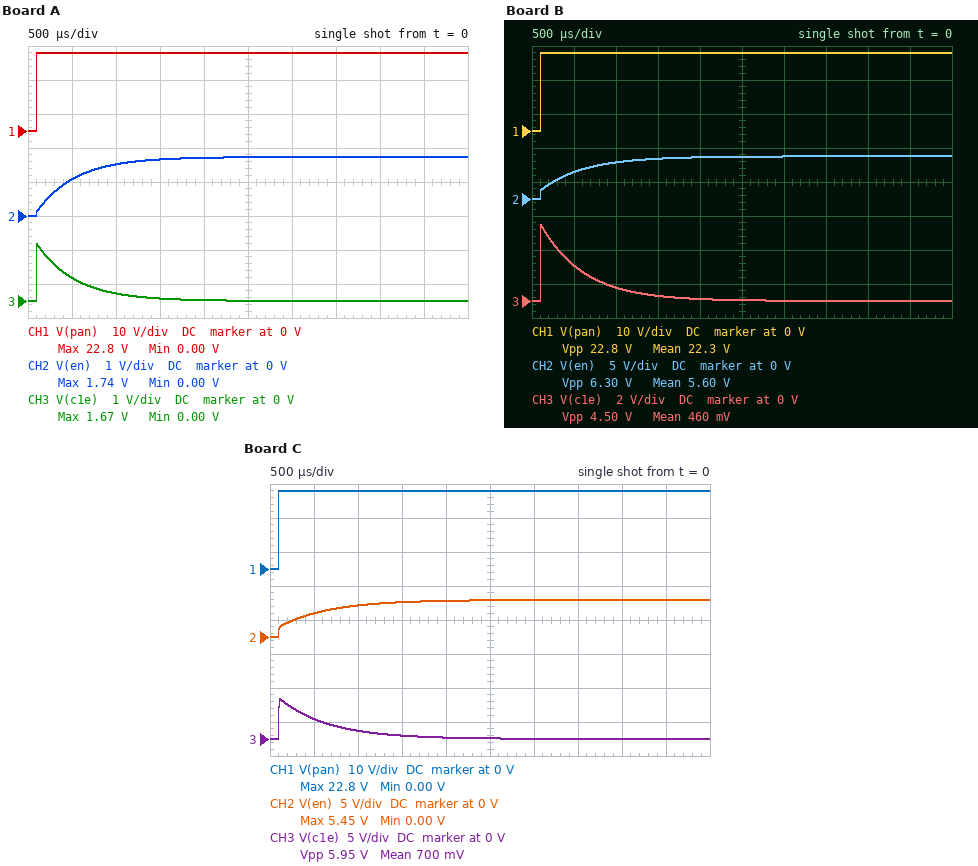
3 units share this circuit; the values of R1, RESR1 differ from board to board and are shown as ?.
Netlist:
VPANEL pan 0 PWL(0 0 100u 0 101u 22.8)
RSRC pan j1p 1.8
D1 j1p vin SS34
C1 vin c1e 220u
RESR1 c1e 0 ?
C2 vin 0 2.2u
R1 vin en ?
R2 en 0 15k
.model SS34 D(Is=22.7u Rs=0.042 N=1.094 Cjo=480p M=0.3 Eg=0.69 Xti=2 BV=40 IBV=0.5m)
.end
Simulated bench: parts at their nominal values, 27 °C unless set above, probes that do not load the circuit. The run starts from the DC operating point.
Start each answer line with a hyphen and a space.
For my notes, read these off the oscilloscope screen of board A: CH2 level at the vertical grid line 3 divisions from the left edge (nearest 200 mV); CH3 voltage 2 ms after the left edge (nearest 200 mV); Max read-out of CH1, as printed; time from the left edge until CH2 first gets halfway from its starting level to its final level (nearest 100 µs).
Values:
- 1.6 V
- 0 V
- 22.8 V
- 400 µs
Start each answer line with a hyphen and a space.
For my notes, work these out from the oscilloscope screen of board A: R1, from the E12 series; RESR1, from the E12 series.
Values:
- 180 kΩ
- 0.15 Ω
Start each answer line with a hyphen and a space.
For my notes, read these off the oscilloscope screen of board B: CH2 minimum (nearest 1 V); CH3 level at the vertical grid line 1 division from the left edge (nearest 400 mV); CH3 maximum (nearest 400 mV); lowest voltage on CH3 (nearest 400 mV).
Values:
- 0 V
- 2.0 V
- 4.4 V
- 0 V
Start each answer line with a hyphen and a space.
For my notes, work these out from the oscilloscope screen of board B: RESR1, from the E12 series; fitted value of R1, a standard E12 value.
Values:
- 0.47 Ω
- 39 kΩ
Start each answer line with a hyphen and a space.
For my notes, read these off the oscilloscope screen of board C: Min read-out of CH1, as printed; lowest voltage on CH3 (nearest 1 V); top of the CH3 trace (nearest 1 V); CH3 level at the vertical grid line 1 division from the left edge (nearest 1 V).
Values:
- 0.00 V
- 0 V
- 6 V
- 3 V
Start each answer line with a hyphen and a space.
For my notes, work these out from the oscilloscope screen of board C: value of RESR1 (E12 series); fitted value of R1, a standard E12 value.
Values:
- 0.68 Ω
- 47 kΩ
